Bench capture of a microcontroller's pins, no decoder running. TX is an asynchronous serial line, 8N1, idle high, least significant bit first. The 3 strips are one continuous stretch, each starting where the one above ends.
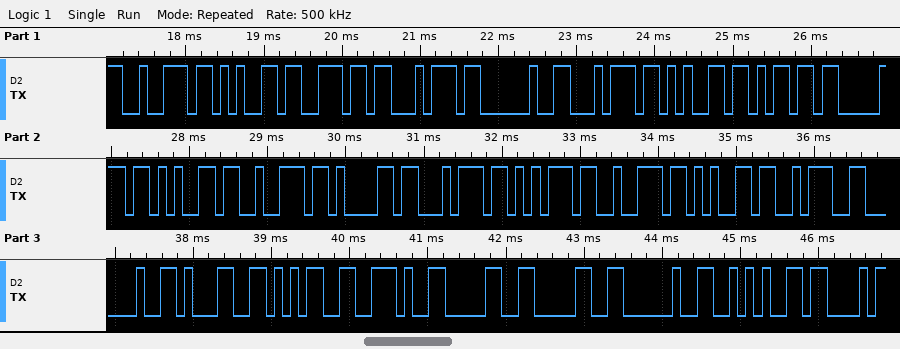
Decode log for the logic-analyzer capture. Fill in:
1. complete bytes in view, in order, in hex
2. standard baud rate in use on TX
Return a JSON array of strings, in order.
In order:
["72 65 6E 74 20 74 65 6D 70 65 72 61 74 75 72 65 3A 20 31 35 2E 30 30 20 2A 43", "9600 baud"]
